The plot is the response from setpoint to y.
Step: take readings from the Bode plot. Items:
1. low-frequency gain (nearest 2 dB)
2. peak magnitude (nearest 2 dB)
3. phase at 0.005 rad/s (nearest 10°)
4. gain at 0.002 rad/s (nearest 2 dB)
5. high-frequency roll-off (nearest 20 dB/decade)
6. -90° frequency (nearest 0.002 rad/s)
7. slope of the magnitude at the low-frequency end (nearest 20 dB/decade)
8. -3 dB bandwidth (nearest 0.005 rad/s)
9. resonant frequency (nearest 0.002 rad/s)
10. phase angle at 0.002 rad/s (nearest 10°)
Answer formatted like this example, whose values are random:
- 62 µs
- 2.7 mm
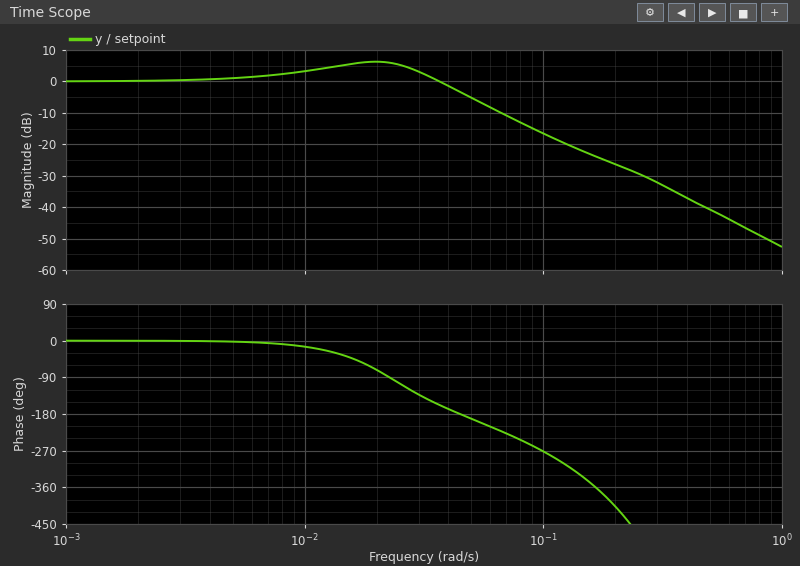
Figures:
- 0 dB
- 6 dB
- 0°
- 0 dB
- -40 dB/decade
- 0.022 rad/s
- 0 dB/decade
- 0.045 rad/s
- 0.020 rad/s
- 0°
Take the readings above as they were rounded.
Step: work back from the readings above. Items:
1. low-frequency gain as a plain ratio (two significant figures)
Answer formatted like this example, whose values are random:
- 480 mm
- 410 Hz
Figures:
- 1.0
